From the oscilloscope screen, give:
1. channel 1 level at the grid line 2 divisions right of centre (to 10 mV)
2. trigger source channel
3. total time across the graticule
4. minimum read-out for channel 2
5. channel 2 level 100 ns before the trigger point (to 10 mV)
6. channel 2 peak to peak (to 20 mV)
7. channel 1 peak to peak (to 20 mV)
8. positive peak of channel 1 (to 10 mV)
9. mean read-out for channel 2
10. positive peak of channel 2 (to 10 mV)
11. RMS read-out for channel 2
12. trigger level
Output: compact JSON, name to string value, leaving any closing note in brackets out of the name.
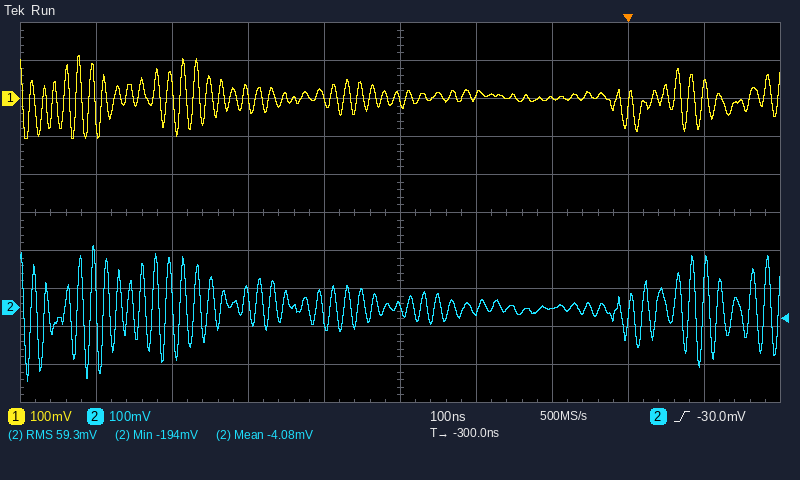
{"channel 1 level at the grid line 2 divisions right of centre": "0 mV", "trigger source channel": "channel 2", "total time across the graticule": "1 µs", "minimum read-out for channel 2": "-194 mV", "channel 2 level 100 ns before the trigger point": "0 mV", "channel 2 peak to peak": "360 mV", "channel 1 peak to peak": "220 mV", "positive peak of channel 1": "110 mV", "mean read-out for channel 2": "-4.08 mV", "positive peak of channel 2": "160 mV", "RMS read-out for channel 2": "59.3 mV", "trigger level": "-30.0 mV"}
